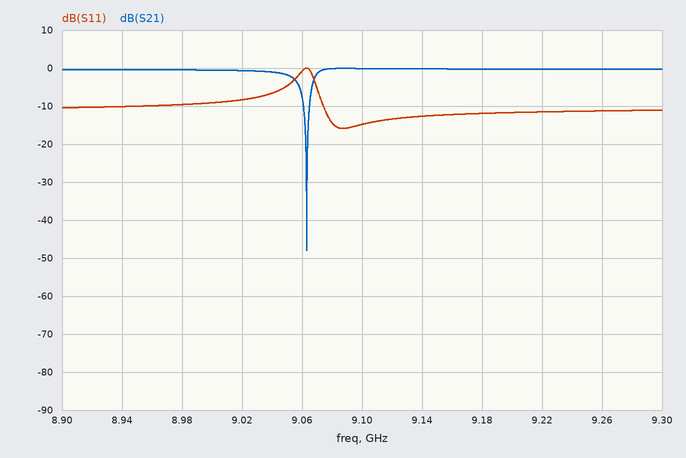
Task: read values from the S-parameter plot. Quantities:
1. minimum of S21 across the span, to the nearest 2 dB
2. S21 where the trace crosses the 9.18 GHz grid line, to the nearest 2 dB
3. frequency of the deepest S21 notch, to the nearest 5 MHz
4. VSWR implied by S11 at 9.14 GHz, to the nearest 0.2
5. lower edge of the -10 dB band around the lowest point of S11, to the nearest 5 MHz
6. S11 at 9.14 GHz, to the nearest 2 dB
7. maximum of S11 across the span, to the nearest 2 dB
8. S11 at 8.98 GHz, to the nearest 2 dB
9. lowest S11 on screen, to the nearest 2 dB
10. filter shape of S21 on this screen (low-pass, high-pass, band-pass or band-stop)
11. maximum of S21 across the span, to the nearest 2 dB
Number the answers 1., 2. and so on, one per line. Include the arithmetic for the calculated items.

1. -48 dB
2. 0 dB
3. 9.065 GHz
4. |Γ| = 10^(-12/20) = 0.2512; VSWR = (1 + 0.2512)/(1 − 0.2512) ≈ 1.67, so 1.6 to the nearest 0.2
5. 9.075 GHz
6. -12 dB
7. 0 dB
8. -10 dB
9. -16 dB
10. band-stop
11. 0 dB
